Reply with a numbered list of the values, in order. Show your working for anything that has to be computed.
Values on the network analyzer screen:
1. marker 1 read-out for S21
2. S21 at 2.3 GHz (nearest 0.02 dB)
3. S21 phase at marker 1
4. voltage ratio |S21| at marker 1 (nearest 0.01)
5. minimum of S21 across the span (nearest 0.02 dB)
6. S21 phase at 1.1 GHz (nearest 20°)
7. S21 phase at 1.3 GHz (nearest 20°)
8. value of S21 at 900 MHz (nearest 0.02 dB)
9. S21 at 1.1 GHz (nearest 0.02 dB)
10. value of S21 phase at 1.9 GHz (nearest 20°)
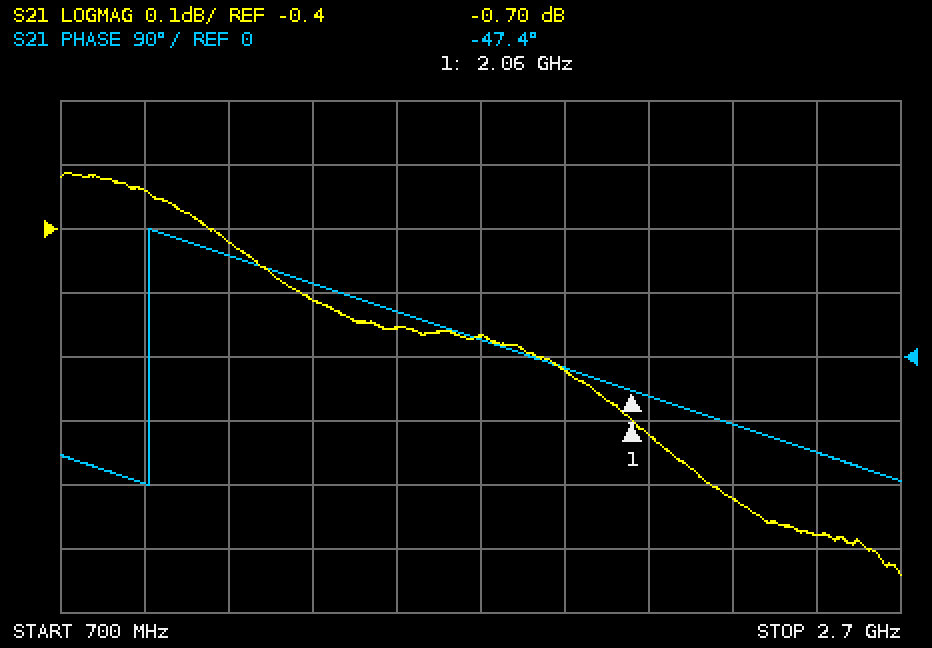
1. -0.70 dB
2. -0.82 dB
3. -47.4°
4. 10^(-0.7/20) ≈ 0.92
5. -0.94 dB
6. 140°
7. 100°
8. -0.34 dB
9. -0.42 dB
10. -20°
